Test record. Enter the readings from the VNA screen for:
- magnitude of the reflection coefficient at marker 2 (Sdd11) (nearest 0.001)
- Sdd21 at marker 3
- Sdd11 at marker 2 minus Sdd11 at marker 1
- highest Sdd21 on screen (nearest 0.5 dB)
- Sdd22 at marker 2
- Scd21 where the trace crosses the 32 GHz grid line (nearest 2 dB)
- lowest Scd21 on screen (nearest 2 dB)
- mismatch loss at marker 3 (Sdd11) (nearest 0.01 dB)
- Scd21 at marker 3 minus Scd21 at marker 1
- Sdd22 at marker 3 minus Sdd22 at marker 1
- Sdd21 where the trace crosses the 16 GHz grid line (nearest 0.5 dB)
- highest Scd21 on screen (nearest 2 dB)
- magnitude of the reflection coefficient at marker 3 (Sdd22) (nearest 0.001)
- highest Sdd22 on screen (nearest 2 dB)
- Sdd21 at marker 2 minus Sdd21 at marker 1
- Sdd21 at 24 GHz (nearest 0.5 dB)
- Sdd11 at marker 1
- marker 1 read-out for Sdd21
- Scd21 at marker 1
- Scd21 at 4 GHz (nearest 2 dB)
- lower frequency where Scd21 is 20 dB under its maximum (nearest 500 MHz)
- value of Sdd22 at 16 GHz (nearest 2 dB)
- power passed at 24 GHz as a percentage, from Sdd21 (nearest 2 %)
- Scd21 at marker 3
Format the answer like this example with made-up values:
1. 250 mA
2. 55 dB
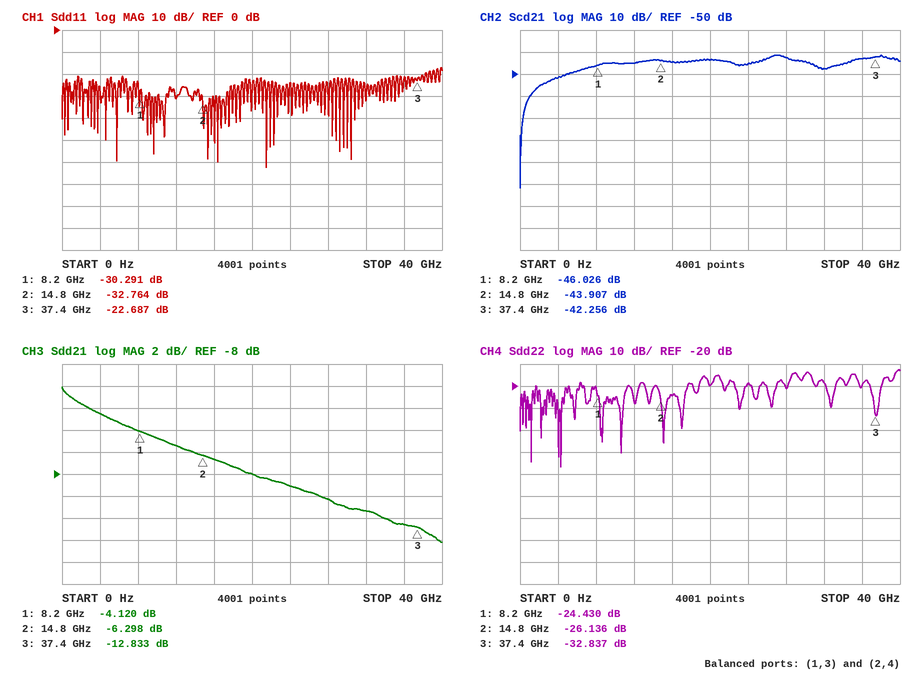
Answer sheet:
1. 0.023
2. -12.833 dB
3. -2.473 dB
4. 0.0 dB
5. -26.136 dB
6. -48 dB
7. -102 dB
8. 0.02 dB
9. 3.770 dB
10. -8.407 dB
11. -6.5 dB
12. -42 dB
13. 0.023
14. -12 dB
15. -2.178 dB
16. -9.0 dB
17. -30.291 dB
18. -4.120 dB
19. -46.026 dB
20. -52 dB
21. 1.0 GHz
22. -24 dB
23. 12 %
24. -42.256 dB
